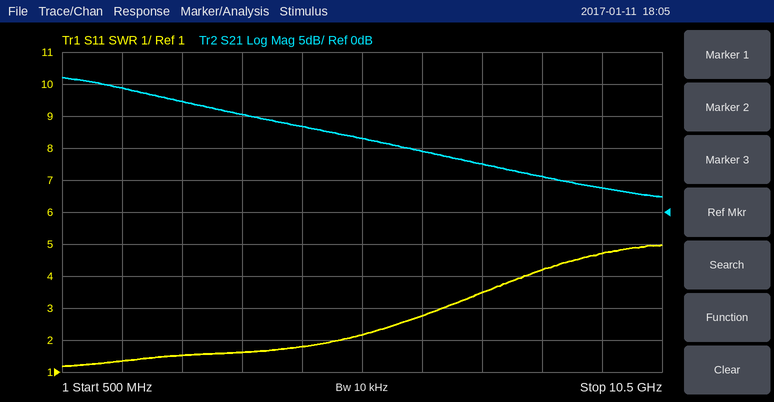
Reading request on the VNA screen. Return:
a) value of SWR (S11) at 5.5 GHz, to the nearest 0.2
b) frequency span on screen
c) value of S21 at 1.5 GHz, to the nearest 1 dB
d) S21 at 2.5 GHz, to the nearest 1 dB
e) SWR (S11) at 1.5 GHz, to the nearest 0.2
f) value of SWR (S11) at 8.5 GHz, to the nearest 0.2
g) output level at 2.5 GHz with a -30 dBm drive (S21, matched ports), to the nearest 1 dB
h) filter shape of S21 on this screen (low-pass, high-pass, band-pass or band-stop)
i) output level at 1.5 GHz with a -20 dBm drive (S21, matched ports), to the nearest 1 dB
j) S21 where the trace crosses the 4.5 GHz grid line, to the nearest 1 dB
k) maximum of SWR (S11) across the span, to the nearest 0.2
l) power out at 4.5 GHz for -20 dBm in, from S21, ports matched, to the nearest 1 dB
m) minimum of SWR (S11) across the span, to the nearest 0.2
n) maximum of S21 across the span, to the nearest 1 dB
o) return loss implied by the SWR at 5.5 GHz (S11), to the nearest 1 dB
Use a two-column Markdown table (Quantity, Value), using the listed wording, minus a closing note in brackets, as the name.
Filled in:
| Quantity | Value |
|---|---|
| value of SWR (S11) at 5.5 GHz, to the nearest 0.2 | 2.2 |
| frequency span on screen | 10 GHz |
| value of S21 at 1.5 GHz, to the nearest 1 dB | 19 dB |
| S21 at 2.5 GHz, to the nearest 1 dB | 17 dB |
| SWR (S11) at 1.5 GHz, to the nearest 0.2 | 1.4 |
| value of SWR (S11) at 8.5 GHz, to the nearest 0.2 | 4.2 |
| output level at 2.5 GHz with a -30 dBm drive (S21, matched ports), to the nearest 1 dB | -13 dBm |
| filter shape of S21 on this screen | low-pass |
| output level at 1.5 GHz with a -20 dBm drive (S21, matched ports), to the nearest 1 dB | -1 dBm |
| S21 where the trace crosses the 4.5 GHz grid line, to the nearest 1 dB | 13 dB |
| maximum of SWR (S11) across the span, to the nearest 0.2 | 5.0 |
| power out at 4.5 GHz for -20 dBm in, from S21, ports matched, to the nearest 1 dB | -7 dBm |
| minimum of SWR (S11) across the span, to the nearest 0.2 | 1.2 |
| maximum of S21 across the span, to the nearest 1 dB | 21 dB |
| return loss implied by the SWR at 5.5 GHz (S11), to the nearest 1 dB | 9 dB |
